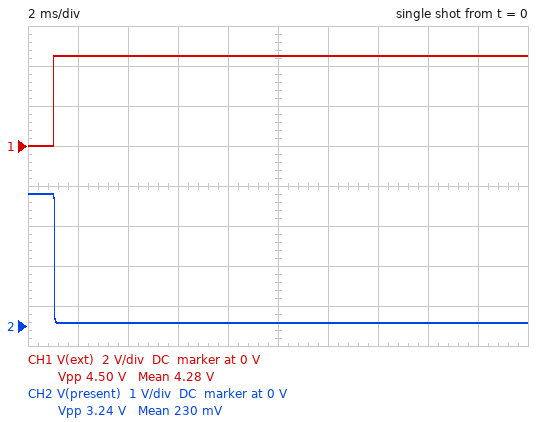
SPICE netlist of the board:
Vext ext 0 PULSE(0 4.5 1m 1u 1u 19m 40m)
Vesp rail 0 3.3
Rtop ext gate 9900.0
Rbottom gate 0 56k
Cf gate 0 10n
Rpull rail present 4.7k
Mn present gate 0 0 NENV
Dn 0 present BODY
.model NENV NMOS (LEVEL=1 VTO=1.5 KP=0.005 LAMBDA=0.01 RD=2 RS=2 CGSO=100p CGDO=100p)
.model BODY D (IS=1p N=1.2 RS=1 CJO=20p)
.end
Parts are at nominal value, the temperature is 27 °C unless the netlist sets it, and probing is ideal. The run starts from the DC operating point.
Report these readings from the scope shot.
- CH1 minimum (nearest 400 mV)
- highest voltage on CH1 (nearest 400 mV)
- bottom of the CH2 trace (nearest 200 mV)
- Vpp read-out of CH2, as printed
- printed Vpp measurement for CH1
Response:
0 V
4.4 V
0 V
3.24 V
4.50 V
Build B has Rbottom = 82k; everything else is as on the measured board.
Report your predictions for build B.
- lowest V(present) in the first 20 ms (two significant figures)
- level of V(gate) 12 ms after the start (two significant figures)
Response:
58 mV
4.0 V
